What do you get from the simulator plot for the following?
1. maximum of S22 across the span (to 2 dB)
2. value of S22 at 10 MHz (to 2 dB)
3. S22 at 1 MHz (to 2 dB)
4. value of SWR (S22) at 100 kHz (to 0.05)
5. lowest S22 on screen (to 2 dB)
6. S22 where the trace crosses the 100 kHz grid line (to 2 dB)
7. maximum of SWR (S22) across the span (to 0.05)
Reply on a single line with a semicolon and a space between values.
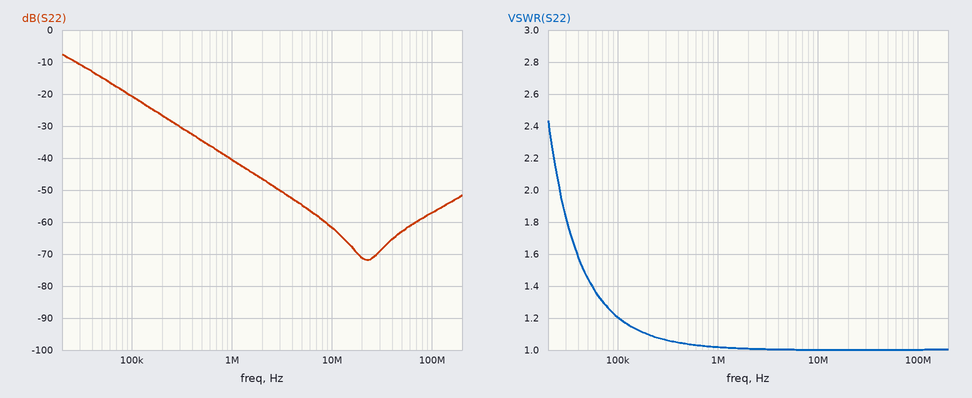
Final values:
-8 dB; -62 dB; -40 dB; 1.20; -72 dB; -20 dB; 2.45
